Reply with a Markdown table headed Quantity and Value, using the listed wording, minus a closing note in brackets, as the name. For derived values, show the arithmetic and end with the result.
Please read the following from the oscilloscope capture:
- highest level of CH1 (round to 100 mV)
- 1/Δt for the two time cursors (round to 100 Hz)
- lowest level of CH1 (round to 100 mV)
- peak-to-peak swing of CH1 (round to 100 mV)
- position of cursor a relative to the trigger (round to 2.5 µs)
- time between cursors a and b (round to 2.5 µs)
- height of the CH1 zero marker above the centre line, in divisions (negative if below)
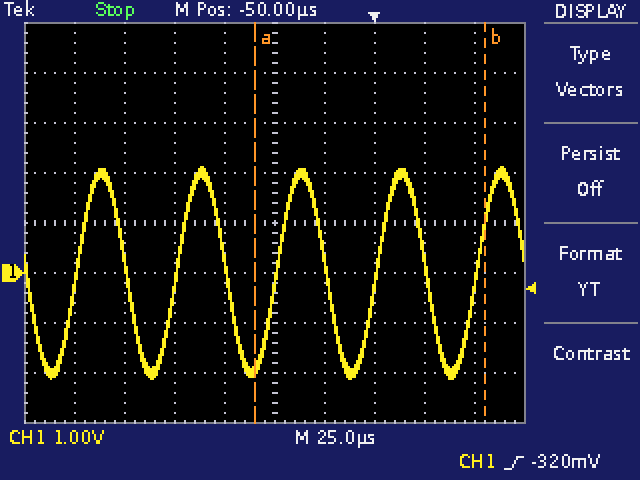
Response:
| Quantity | Value |
|---|---|
| highest level of CH1 | 2.1 V |
| 1/Δt for the two time cursors | 1 / 115.0 µs ≈ 8.7 kHz |
| lowest level of CH1 | -2.1 V |
| peak-to-peak swing of CH1 | 2.1 V − (-2.1 V) = 4.2 V |
| position of cursor a relative to the trigger | -60.0 µs |
| time between cursors a and b | 115.0 µs |
| height of the CH1 zero marker above the centre line, in divisions | -1.0 div |
